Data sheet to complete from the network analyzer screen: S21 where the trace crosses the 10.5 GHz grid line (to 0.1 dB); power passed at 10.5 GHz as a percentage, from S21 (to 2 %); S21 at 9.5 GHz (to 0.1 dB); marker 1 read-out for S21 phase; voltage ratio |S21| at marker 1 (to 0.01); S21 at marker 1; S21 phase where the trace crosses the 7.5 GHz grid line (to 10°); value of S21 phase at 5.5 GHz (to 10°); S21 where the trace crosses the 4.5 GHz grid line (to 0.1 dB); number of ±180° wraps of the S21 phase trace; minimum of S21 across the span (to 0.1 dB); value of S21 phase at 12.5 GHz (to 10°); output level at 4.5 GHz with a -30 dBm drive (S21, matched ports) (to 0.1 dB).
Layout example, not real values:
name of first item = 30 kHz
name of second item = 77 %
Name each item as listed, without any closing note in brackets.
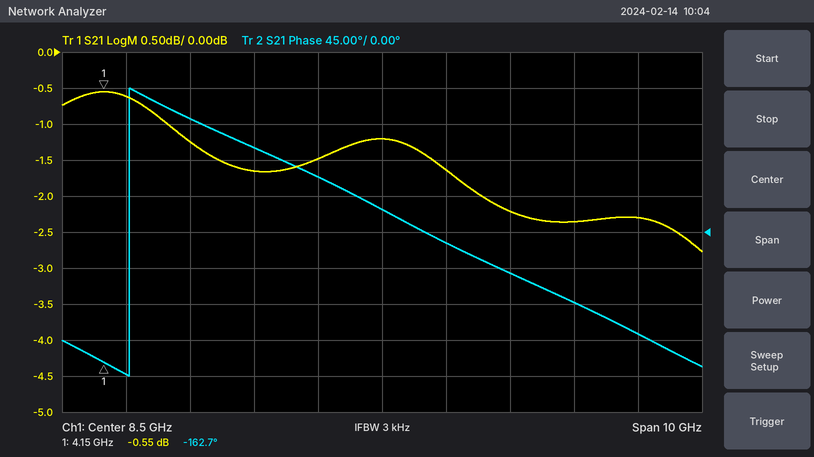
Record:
S21 where the trace crosses the 10.5 GHz grid line = -2.2 dB
power passed at 10.5 GHz as a percentage, from S21 = 60 %
S21 at 9.5 GHz = -1.6 dB
marker 1 read-out for S21 phase = -162.7°
voltage ratio |S21| at marker 1 = 0.94
S21 at marker 1 = -0.55 dB
S21 phase where the trace crosses the 7.5 GHz grid line = 70°
value of S21 phase at 5.5 GHz = 140°
S21 where the trace crosses the 4.5 GHz grid line = -0.6 dB
number of ±180° wraps of the S21 phase trace = 1
minimum of S21 across the span = -2.8 dB
value of S21 phase at 12.5 GHz = -130°
output level at 4.5 GHz with a -30 dBm drive (S21, matched ports) = -30.6 dBm
